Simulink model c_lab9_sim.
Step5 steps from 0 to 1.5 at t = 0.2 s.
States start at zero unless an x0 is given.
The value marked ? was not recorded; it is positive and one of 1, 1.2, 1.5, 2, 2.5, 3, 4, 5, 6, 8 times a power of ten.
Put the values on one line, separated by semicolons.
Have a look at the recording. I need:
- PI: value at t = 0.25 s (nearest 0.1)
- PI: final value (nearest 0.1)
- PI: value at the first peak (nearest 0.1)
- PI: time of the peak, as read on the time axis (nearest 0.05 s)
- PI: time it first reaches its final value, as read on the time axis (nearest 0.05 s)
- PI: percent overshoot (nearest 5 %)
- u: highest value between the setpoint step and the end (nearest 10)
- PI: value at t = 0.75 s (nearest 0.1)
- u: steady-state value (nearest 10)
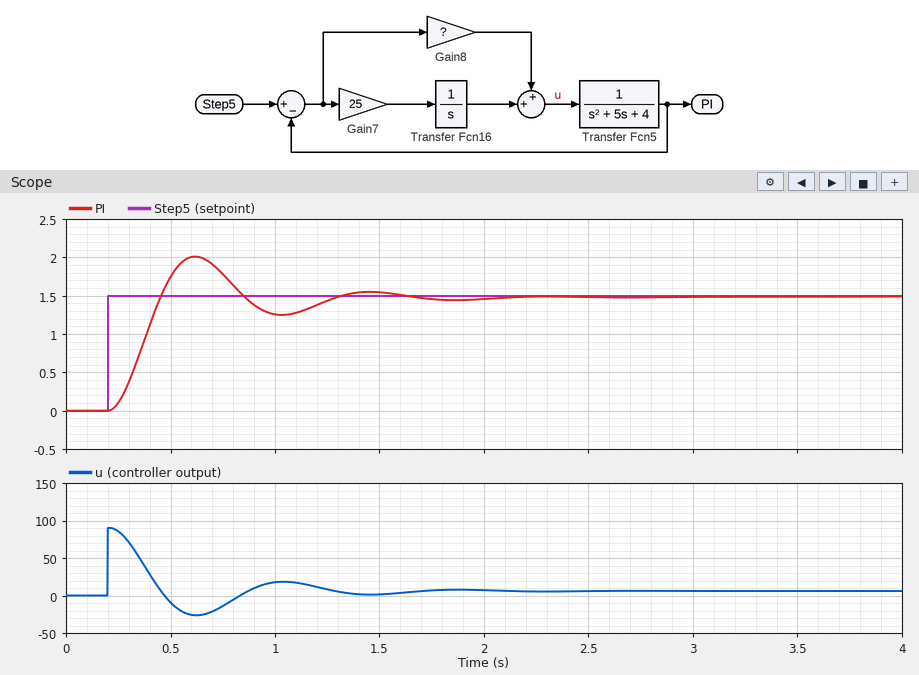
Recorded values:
0.1; 1.5; 2.0; 0.60 s; 0.45 s; 35 %; 90; 1.8; 10
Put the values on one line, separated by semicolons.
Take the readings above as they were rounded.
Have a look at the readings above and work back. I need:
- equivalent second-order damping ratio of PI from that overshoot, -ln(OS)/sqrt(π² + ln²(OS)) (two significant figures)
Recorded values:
0.32
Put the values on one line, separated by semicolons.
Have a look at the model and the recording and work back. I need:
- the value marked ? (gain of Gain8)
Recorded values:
60
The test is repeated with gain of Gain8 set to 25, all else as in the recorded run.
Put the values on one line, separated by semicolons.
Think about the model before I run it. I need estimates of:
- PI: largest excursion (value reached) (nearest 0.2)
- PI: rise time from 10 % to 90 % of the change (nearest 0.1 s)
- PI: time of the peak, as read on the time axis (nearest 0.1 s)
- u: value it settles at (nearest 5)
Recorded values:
1.8; 0.3 s; 0.9 s; 5
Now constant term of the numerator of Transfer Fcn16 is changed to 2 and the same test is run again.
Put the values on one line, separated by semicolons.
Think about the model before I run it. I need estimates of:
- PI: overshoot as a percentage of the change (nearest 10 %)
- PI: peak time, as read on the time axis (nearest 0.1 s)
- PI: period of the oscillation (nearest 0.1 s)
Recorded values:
40 %; 0.6 s; 0.8 s
